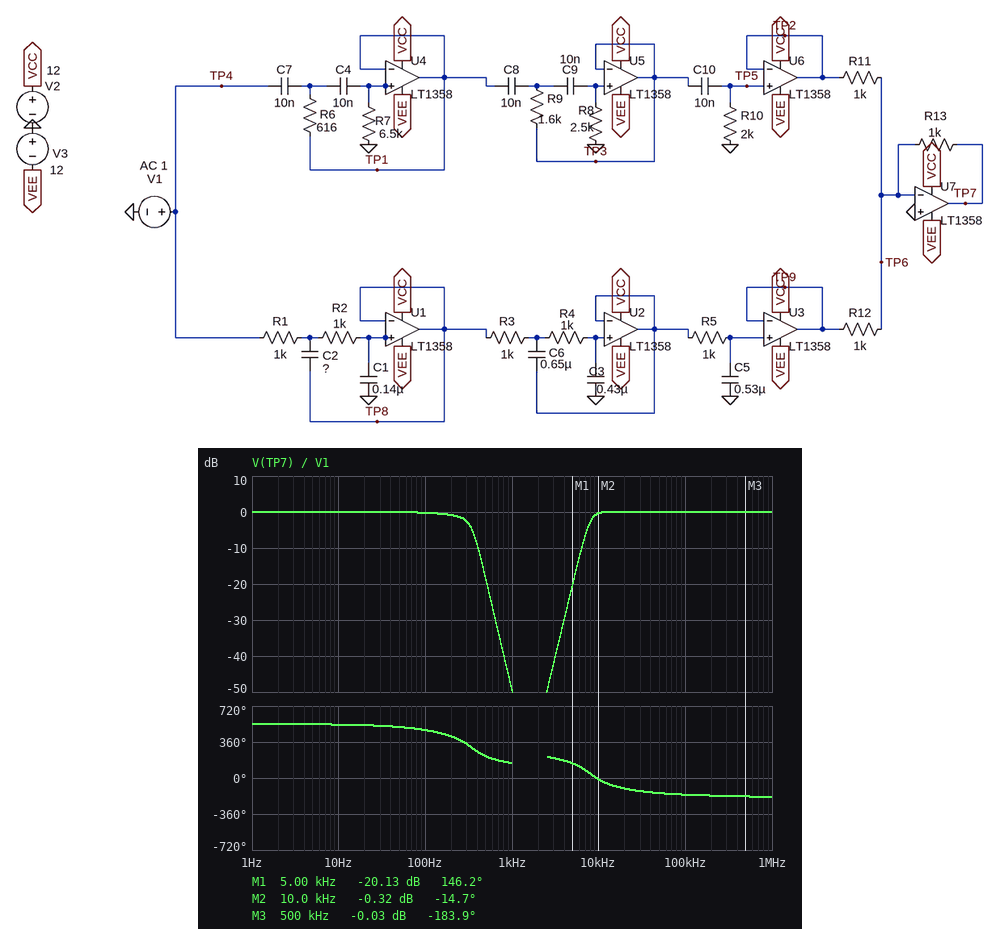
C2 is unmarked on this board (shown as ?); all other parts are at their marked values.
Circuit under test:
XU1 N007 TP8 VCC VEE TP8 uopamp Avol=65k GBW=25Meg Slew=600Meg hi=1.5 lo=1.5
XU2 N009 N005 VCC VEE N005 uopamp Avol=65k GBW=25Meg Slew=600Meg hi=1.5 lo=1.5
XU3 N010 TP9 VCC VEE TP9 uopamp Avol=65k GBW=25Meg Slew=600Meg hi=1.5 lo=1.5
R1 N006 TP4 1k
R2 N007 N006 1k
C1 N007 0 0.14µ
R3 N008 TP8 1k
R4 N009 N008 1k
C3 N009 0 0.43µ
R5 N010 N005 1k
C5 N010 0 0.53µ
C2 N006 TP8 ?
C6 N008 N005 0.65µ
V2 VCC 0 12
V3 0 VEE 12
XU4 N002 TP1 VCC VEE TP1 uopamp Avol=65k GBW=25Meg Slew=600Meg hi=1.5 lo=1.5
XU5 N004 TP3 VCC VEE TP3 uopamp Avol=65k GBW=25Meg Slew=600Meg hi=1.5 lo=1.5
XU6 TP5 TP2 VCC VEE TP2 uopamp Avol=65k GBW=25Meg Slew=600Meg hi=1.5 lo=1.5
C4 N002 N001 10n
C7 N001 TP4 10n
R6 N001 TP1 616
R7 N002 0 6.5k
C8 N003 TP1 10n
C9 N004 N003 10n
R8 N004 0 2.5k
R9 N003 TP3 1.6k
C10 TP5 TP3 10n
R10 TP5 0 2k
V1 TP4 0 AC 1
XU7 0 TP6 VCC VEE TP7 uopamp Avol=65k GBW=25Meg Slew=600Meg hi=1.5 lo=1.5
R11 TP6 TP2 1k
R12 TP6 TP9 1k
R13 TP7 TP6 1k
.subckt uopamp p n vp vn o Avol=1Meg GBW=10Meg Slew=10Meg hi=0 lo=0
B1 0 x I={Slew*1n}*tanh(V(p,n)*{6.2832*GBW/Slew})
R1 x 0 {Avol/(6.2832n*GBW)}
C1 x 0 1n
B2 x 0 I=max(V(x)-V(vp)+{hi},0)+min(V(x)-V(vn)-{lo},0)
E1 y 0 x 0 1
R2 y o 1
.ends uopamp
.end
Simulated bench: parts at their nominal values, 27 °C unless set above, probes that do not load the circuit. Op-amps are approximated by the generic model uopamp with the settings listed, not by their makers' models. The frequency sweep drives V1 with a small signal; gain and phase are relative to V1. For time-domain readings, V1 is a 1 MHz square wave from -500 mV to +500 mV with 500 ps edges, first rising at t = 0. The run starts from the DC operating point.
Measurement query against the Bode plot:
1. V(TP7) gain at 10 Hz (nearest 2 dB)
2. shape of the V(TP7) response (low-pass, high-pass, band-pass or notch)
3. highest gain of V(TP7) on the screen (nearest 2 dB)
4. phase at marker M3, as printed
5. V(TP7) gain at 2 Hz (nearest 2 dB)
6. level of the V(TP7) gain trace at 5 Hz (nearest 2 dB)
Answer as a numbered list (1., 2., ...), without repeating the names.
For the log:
1. 0 dB
2. notch
3. 0 dB
4. -183.9 deg
5. 0 dB
6. 0 dB
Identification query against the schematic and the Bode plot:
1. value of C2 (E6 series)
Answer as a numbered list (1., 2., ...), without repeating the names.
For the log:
1. 1.5 µF
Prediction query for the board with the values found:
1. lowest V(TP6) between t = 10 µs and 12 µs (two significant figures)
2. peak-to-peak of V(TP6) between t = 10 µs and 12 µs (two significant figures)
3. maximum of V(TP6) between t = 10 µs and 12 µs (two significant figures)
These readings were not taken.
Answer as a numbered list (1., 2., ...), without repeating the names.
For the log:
1. -150 mV
2. 300 mV
3. 150 mV
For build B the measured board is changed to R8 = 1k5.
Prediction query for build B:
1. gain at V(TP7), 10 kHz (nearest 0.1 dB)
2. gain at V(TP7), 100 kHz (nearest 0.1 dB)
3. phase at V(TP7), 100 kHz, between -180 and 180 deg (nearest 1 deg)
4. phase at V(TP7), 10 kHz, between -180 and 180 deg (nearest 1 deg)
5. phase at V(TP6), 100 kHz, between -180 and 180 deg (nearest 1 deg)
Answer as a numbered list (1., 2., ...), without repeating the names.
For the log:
1. -4.4 dB
2. -0.1 dB
3. -162 deg
4. 3 deg
5. 108 deg
